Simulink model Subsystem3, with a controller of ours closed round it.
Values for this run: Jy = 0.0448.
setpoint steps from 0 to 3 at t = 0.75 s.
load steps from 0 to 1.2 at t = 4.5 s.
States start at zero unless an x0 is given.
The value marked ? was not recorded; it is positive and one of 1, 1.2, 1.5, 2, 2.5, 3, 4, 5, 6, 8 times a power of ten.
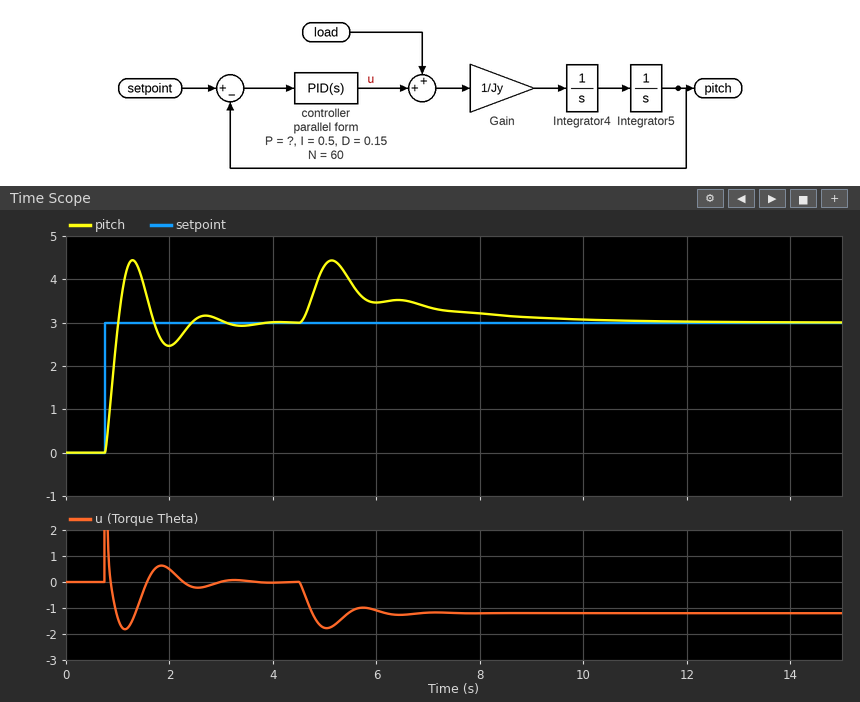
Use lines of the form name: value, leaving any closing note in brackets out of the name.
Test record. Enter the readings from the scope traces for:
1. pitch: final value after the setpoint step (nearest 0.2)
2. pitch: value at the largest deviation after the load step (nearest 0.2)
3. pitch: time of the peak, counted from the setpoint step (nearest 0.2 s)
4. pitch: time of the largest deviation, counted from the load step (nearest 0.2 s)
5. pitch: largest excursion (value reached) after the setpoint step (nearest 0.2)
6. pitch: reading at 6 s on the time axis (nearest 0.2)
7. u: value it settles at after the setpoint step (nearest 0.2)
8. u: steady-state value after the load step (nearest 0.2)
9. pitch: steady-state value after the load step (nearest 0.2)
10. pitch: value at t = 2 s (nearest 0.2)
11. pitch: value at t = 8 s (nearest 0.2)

pitch: final value after the setpoint step: 3.0
pitch: value at the largest deviation after the load step: 4.4
pitch: time of the peak, counted from the setpoint step: 0.6 s
pitch: time of the largest deviation, counted from the load step: 0.6 s
pitch: largest excursion (value reached) after the setpoint step: 4.4
pitch: reading at 6 s on the time axis: 3.4
u: value it settles at after the setpoint step: 0.0
u: steady-state value after the load step: -1.2
pitch: steady-state value after the load step: 3.0
pitch: value at t = 2 s: 2.4
pitch: value at t = 8 s: 3.2
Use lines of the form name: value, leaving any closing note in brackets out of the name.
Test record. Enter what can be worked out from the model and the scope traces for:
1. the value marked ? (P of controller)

the value marked ?: 1
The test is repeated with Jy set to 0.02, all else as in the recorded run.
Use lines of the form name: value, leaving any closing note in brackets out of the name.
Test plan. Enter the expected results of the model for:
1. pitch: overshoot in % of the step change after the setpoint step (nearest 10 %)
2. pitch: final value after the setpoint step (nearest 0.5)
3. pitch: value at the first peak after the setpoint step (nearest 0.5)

pitch: overshoot in % of the step change after the setpoint step: 30 %
pitch: final value after the setpoint step: 3.0
pitch: value at the first peak after the setpoint step: 4.0
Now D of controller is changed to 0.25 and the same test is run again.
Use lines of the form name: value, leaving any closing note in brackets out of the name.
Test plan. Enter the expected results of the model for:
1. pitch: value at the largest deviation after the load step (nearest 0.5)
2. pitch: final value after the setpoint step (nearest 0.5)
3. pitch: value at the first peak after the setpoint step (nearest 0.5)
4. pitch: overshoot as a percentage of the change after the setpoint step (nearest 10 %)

pitch: value at the largest deviation after the load step: 4.0
pitch: final value after the setpoint step: 3.0
pitch: value at the first peak after the setpoint step: 4.0
pitch: overshoot as a percentage of the change after the setpoint step: 30 %
